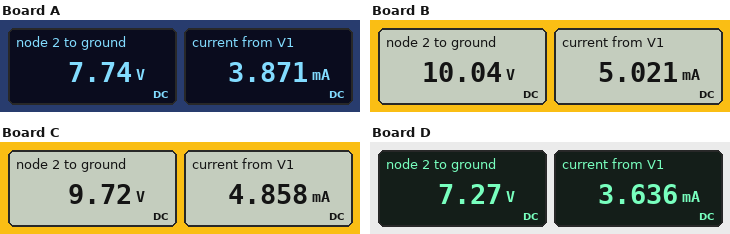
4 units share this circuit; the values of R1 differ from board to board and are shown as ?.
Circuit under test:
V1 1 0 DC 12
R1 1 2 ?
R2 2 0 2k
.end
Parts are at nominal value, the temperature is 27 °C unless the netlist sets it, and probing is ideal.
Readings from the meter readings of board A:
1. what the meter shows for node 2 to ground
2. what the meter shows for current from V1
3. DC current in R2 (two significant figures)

7.74 V
3.871 mA
3.9 mA
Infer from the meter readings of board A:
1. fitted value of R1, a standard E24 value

1.1 kΩ
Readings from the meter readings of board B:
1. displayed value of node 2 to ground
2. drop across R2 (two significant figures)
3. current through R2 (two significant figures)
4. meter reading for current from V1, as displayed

10.04 V
10 V
5.0 mA
5.021 mA
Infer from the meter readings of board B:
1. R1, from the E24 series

390 Ω
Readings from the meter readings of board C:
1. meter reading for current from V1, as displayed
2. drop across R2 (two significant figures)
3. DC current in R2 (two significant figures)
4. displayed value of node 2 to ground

4.858 mA
9.7 V
4.9 mA
9.72 V
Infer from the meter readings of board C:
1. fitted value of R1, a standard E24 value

470 Ω
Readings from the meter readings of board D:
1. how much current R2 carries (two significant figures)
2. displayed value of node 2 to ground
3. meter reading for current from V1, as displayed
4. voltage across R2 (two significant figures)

3.6 mA
7.27 V
3.636 mA
7.3 V
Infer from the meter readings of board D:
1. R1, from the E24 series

1.3 kΩ
